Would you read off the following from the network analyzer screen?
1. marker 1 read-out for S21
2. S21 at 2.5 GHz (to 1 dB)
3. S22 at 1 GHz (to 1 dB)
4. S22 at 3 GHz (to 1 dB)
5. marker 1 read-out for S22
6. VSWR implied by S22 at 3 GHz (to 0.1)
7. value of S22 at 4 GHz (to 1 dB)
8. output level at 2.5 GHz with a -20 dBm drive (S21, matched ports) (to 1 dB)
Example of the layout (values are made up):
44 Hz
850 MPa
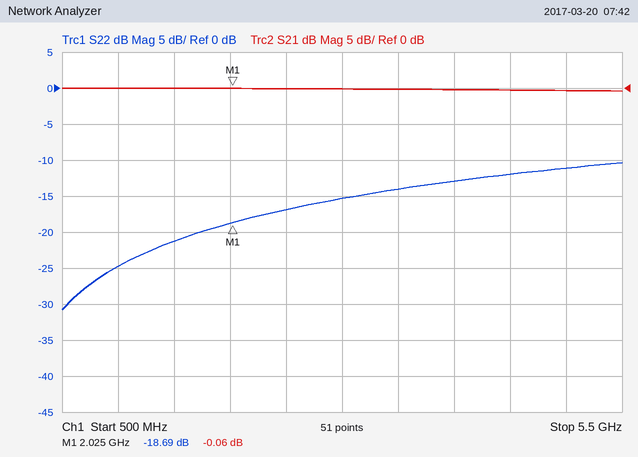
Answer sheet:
-0.06 dB
0 dB
-25 dB
-15 dB
-18.69 dB
1.4
-13 dB
-20 dBm
